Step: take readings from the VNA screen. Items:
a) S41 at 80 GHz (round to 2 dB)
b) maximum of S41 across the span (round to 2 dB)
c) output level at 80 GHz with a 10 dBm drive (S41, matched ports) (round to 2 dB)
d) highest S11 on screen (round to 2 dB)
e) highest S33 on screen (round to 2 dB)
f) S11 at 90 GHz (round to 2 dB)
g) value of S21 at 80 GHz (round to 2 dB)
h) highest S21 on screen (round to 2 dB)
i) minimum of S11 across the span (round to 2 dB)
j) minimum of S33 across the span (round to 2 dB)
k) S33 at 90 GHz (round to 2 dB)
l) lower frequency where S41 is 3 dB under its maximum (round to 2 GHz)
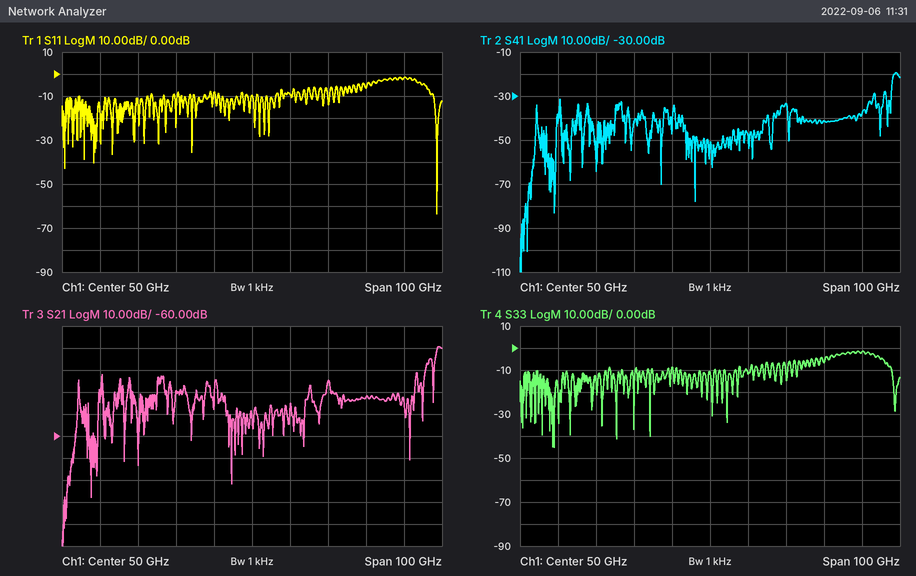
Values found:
-42 dB
-20 dB
-32 dBm
-2 dB
-2 dB
-2 dB
-42 dB
-20 dB
-64 dB
-46 dB
-2 dB
98 GHz
